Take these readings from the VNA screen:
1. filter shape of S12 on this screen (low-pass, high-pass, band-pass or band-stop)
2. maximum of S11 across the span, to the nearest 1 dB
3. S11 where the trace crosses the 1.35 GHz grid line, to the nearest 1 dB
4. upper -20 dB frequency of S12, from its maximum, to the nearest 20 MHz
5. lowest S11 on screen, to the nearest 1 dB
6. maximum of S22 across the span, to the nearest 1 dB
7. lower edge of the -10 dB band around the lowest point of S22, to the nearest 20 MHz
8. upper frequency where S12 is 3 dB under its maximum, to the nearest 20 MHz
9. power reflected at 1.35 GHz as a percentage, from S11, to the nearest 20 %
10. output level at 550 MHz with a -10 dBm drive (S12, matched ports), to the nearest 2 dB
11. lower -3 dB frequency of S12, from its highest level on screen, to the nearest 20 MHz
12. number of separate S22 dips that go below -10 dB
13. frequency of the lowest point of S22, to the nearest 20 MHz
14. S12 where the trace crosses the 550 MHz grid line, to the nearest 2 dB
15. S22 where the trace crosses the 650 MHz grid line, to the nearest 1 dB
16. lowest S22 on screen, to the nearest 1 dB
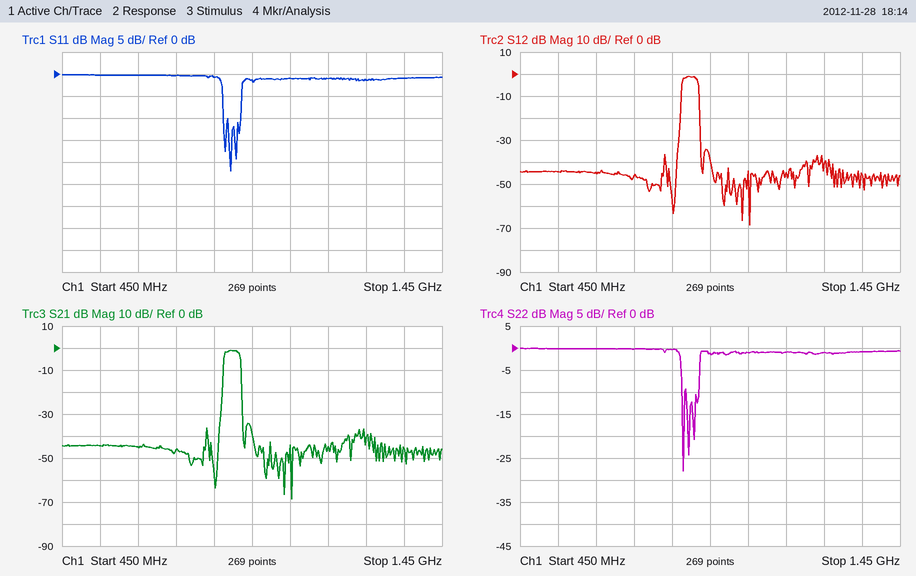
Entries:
band-pass
0 dB
-1 dB
920 MHz
-22 dB
0 dB
880 MHz
920 MHz
80 %
-54 dBm
880 MHz
3
880 MHz
-44 dB
0 dB
-28 dB
